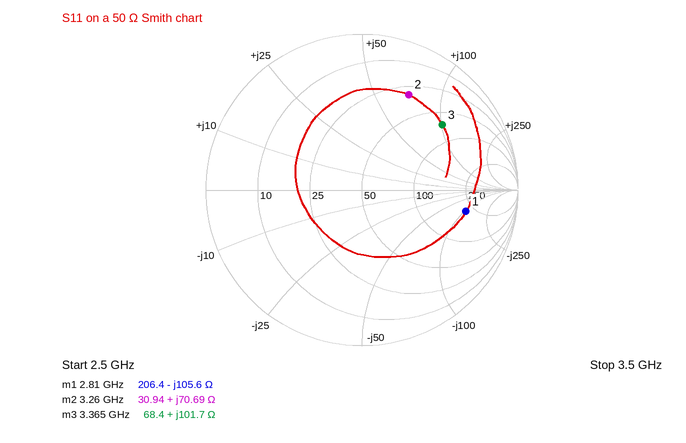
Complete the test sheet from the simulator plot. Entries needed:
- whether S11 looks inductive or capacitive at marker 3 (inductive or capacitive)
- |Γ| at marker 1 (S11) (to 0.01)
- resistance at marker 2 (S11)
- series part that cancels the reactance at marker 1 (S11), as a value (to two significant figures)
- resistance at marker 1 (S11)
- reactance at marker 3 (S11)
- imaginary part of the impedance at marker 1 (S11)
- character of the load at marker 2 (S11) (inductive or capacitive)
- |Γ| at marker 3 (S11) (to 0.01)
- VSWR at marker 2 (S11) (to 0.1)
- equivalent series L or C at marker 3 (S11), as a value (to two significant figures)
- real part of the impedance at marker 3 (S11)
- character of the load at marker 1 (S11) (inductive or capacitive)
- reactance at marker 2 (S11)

inductive
0.68
30.94 Ω
6.0 nH
206.4 Ω
+101.7 Ω
-105.6 Ω
inductive
0.66
5.3
4.8 nH
68.4 Ω
capacitive
+70.69 Ω
